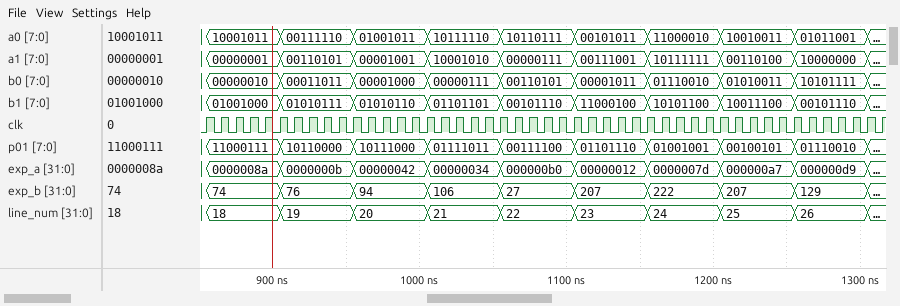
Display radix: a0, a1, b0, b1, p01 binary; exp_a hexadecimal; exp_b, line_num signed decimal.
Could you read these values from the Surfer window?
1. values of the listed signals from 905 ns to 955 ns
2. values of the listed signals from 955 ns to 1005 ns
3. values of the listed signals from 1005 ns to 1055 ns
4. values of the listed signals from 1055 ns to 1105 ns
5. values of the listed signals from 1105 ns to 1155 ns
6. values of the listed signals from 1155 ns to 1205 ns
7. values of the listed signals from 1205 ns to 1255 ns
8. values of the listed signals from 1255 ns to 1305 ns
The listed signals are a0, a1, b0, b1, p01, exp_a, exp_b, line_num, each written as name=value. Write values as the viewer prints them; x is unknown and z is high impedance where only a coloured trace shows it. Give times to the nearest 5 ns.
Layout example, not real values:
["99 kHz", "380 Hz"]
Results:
["a0=00111110, a1=00110101, b0=00011011, b1=01010111, p01=10110000, exp_a=0000000b, exp_b=76, line_num=19", "a0=01001011, a1=00001001, b0=00001000, b1=01010110, p01=10111000, exp_a=00000042, exp_b=94, line_num=20", "a0=10111110, a1=10001010, b0=00000111, b1=01101101, p01=01111011, exp_a=00000034, exp_b=106, line_num=21", "a0=10110111, a1=00000111, b0=00110101, b1=00101110, p01=00111100, exp_a=000000b0, exp_b=27, line_num=22", "a0=00101011, a1=00111001, b0=00001011, b1=11000100, p01=01101110, exp_a=00000012, exp_b=207, line_num=23", "a0=11000010, a1=10111111, b0=01110010, b1=10101100, p01=01001001, exp_a=0000007d, exp_b=222, line_num=24", "a0=10010011, a1=00110100, b0=01010011, b1=10011100, p01=00100101, exp_a=000000a7, exp_b=207, line_num=25", "a0=01011001, a1=10000000, b0=10101111, b1=00101110, p01=01110010, exp_a=000000d9, exp_b=129, line_num=26"]
